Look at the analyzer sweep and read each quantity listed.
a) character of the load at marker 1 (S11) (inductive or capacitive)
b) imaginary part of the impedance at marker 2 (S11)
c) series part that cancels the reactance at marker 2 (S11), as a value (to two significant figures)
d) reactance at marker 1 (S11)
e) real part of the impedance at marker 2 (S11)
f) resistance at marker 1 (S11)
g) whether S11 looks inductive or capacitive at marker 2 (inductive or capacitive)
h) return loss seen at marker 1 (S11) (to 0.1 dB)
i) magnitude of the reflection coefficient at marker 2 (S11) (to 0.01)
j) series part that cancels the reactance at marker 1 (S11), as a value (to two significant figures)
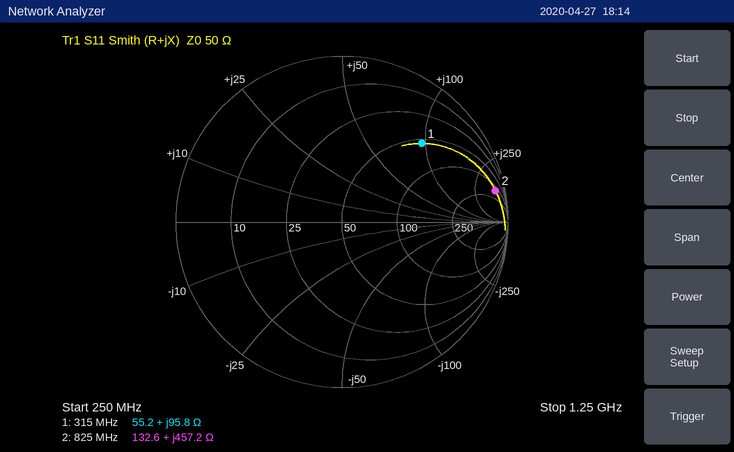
inductive
+457.2 Ω
420 fF
+95.8 Ω
132.6 Ω
55.2 Ω
inductive
3.4 dB
0.94
5.3 pF
